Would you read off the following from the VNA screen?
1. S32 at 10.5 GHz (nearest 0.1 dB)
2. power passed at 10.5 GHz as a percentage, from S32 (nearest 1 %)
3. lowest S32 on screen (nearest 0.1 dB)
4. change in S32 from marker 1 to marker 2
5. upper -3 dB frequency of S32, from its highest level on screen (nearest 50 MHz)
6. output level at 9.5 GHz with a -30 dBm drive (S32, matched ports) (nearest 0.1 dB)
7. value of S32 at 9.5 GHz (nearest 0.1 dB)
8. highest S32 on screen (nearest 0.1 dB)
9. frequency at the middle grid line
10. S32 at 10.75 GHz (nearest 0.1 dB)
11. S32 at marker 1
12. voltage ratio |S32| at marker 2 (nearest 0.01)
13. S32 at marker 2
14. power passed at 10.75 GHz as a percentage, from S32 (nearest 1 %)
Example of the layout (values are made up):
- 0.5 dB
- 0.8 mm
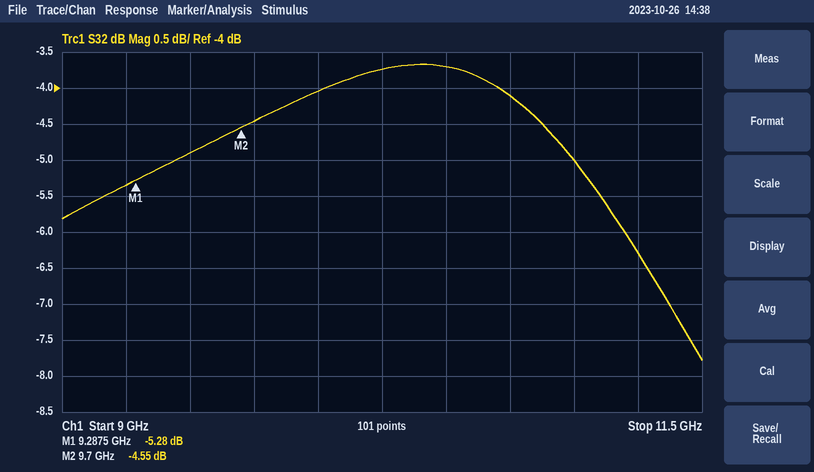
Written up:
- -3.7 dB
- 43 %
- -7.8 dB
- 0.73 dB
- 11.30 GHz
- -34.9 dBm
- -4.9 dB
- -3.7 dB
- 10.25 GHz
- -4.1 dB
- -5.28 dB
- 0.59
- -4.55 dB
- 39 %
